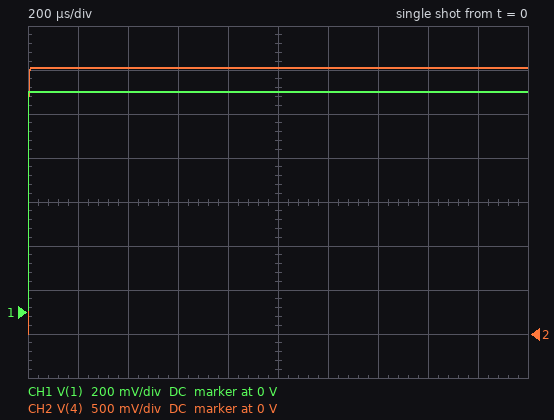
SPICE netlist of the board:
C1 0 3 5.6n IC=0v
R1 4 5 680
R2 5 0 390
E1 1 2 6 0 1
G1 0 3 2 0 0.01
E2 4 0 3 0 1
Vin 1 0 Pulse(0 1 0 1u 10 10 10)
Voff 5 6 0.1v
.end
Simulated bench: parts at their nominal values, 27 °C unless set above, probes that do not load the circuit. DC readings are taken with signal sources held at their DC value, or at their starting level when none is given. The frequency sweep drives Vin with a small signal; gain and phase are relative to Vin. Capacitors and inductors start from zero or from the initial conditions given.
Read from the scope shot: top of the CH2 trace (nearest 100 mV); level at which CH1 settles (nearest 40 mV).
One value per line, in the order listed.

3.0 V
1.00 V
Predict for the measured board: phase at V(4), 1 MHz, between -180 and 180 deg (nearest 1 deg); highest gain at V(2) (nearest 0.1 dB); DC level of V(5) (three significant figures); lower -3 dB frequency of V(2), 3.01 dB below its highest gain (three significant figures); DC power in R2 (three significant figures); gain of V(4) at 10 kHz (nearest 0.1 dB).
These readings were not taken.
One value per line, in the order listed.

-84 deg
0 dB
100 mV
104 kHz
25.6 µW
8.7 dB
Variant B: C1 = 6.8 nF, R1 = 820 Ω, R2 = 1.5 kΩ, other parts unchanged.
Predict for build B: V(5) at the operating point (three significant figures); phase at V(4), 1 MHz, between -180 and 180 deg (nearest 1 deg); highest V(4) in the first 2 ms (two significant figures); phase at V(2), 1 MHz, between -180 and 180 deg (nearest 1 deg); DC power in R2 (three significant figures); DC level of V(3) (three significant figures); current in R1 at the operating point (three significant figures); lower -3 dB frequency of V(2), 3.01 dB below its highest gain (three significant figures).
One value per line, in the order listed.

100 mV
-81 deg
1.7 V
9 deg
6.67 µW
155 mV
66.7 µA
151 kHz
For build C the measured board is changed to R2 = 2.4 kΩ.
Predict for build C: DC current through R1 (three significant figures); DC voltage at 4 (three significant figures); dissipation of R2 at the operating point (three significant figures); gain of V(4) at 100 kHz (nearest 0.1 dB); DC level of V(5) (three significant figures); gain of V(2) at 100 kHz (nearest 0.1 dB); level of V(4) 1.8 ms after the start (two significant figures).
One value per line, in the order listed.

41.7 µA
128 mV
4.17 µW
1.4 dB
100 mV
-7.7 dB
1.4 V
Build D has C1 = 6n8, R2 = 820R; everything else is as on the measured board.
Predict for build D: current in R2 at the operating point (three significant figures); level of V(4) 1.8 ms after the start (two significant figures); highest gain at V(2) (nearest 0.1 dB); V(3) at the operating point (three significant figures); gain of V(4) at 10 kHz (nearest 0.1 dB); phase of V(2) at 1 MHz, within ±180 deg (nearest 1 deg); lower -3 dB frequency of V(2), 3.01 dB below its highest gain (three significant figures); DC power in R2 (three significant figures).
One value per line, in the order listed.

122 µA
2.0 V
0 dB
183 mV
5.2 dB
7 deg
128 kHz
12.2 µW
